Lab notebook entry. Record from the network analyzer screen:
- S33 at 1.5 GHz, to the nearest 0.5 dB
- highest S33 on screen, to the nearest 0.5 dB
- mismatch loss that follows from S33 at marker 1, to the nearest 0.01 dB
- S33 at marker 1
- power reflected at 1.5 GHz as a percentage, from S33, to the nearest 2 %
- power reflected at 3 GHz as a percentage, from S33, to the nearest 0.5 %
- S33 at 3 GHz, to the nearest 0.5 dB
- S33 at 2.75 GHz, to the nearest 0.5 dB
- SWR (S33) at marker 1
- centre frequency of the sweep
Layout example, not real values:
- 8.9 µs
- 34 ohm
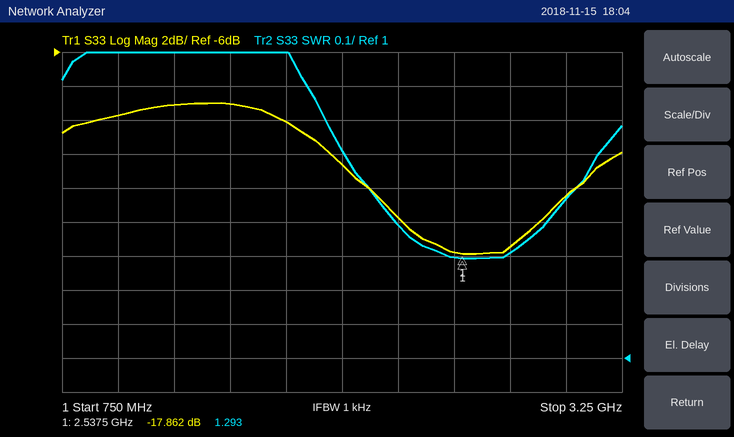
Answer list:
- -9.0 dB
- -9.0 dB
- 0.07 dB
- -17.862 dB
- 12 %
- 3.5 %
- -14.5 dB
- -17.5 dB
- 1.293
- 2 GHz
